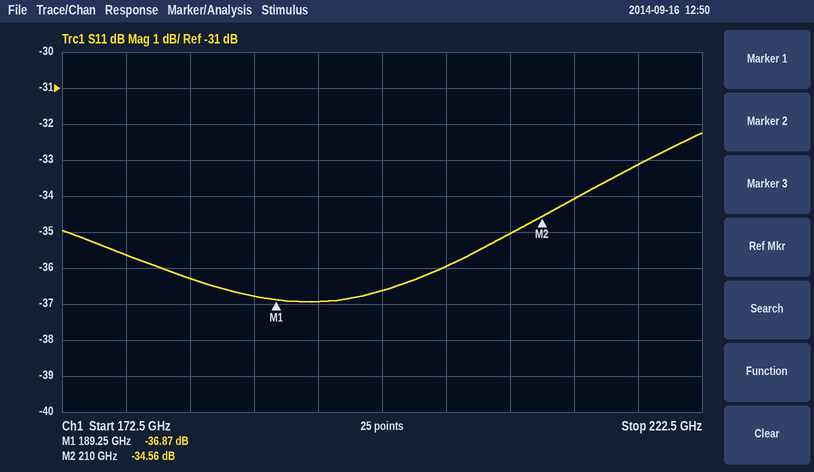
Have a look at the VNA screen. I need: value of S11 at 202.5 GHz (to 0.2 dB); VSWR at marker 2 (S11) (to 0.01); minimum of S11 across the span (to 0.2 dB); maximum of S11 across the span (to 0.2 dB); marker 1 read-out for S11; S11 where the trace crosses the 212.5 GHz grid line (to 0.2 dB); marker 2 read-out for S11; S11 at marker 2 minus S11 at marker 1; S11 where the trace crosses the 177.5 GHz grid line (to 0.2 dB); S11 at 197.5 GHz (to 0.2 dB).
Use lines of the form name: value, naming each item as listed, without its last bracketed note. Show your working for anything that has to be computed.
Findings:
value of S11 at 202.5 GHz: -36.0 dB
VSWR at marker 2 (S11): (1 + 0.0187)/(1 − 0.0187) ≈ 1.04
minimum of S11 across the span: -37.0 dB
maximum of S11 across the span: -32.2 dB
marker 1 read-out for S11: -36.87 dB
S11 where the trace crosses the 212.5 GHz grid line: -34.0 dB
marker 2 read-out for S11: -34.56 dB
S11 at marker 2 minus S11 at marker 1: -34.56 − (-36.87) = 2.31 dB
S11 where the trace crosses the 177.5 GHz grid line: -35.6 dB
S11 at 197.5 GHz: -36.6 dB
